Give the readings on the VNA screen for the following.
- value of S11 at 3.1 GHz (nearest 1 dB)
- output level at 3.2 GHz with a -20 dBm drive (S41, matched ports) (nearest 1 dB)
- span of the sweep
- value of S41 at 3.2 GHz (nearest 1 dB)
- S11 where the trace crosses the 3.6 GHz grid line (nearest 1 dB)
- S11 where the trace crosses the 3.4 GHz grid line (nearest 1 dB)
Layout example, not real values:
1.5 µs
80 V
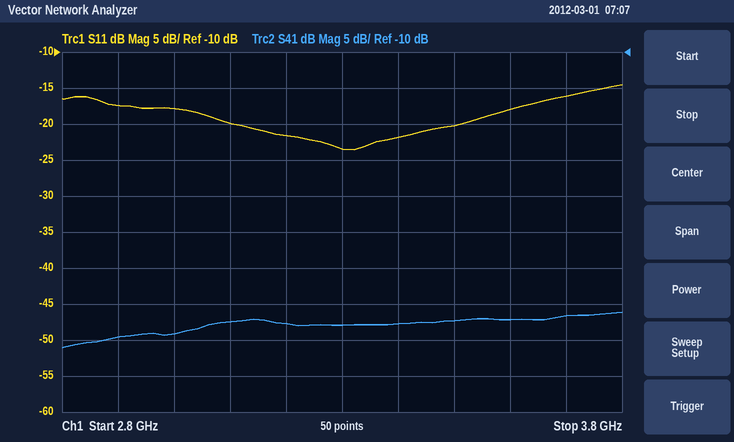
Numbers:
-20 dB
-68 dBm
1 GHz
-48 dB
-18 dB
-22 dB
